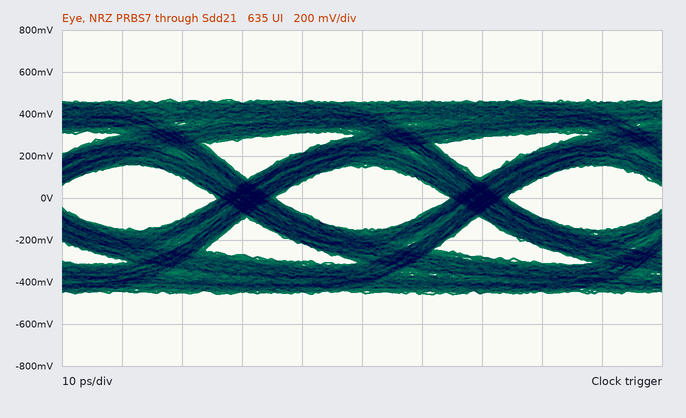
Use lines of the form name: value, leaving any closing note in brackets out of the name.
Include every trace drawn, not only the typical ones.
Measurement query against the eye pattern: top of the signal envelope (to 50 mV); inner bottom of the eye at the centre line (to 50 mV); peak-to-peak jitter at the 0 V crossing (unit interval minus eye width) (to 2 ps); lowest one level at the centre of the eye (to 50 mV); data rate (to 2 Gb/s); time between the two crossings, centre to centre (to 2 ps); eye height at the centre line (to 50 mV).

top of the signal envelope: 450 mV
inner bottom of the eye at the centre line: -150 mV
peak-to-peak jitter at the 0 V crossing (unit interval minus eye width): 10 ps
lowest one level at the centre of the eye: 150 mV
data rate: 26 Gb/s
time between the two crossings, centre to centre: 38 ps
eye height at the centre line: 300 mV
